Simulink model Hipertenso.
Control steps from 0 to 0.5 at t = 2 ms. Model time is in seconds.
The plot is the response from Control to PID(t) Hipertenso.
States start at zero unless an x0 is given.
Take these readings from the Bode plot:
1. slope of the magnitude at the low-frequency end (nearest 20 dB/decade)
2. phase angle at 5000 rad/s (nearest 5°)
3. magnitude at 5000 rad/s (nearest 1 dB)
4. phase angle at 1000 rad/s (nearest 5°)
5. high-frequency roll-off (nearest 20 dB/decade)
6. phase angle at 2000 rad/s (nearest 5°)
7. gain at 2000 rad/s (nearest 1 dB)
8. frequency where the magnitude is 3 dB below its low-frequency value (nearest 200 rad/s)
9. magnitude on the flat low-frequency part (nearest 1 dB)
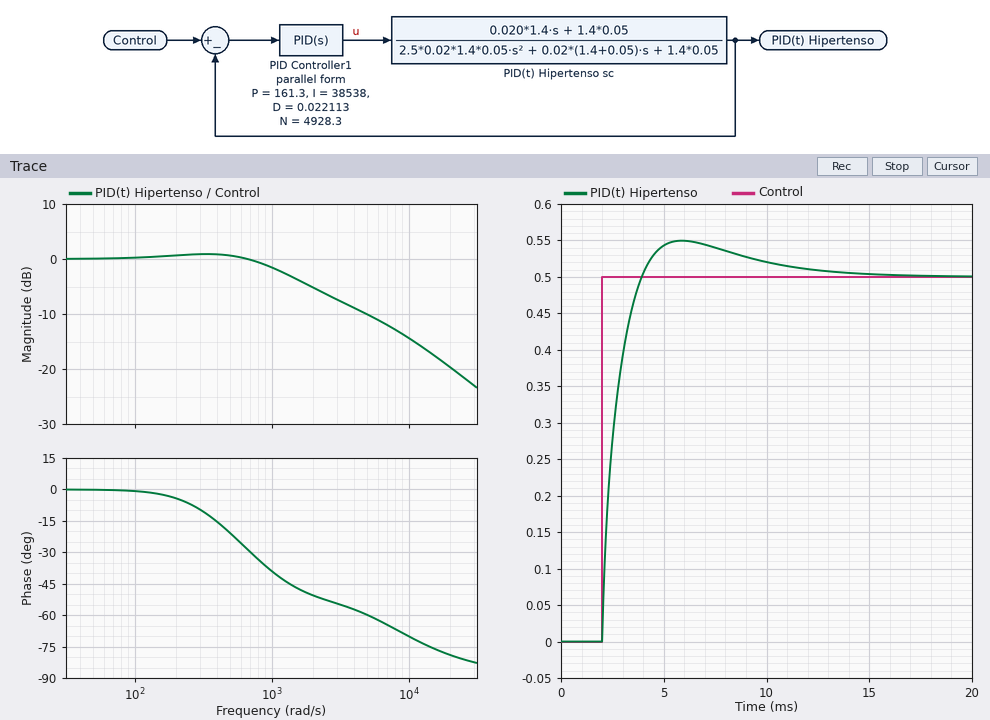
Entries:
0 dB/decade
-60°
-10 dB
-40°
-20 dB/decade
-50°
-5 dB
1400 rad/s
0 dB
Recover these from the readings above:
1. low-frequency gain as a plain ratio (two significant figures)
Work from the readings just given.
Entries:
1.0
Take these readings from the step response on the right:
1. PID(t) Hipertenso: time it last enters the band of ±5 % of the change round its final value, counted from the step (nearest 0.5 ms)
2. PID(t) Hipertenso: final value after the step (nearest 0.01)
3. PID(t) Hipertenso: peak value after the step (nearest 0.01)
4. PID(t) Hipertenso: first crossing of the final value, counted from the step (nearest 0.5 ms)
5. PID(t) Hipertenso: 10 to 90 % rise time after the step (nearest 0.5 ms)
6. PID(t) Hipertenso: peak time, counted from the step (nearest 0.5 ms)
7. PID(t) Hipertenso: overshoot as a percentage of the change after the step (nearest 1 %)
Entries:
7.5 ms
0.50
0.55
2.0 ms
1.5 ms
4.0 ms
10 %
